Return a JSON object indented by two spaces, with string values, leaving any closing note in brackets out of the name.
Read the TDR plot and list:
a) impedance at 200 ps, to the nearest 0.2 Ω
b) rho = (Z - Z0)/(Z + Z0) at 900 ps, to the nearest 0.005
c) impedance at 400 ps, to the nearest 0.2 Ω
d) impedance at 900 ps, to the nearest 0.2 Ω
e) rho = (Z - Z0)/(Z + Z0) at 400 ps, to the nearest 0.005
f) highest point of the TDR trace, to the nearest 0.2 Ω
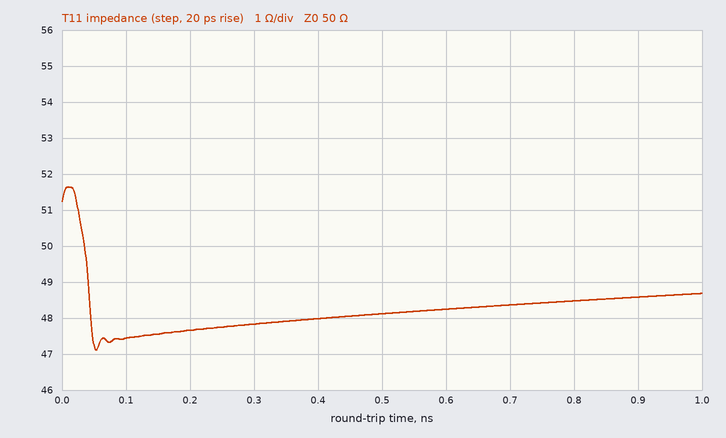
{
  "impedance at 200 ps, to the nearest 0.2 Ω": "47.6 Ω",
  "rho = (Z - Z0)/(Z + Z0) at 900 ps, to the nearest 0.005": "-0.015",
  "impedance at 400 ps, to the nearest 0.2 Ω": "48.0 Ω",
  "impedance at 900 ps, to the nearest 0.2 Ω": "48.6 Ω",
  "rho = (Z - Z0)/(Z + Z0) at 400 ps, to the nearest 0.005": "-0.020",
  "highest point of the TDR trace, to the nearest 0.2 Ω": "51.6 Ω"
}
